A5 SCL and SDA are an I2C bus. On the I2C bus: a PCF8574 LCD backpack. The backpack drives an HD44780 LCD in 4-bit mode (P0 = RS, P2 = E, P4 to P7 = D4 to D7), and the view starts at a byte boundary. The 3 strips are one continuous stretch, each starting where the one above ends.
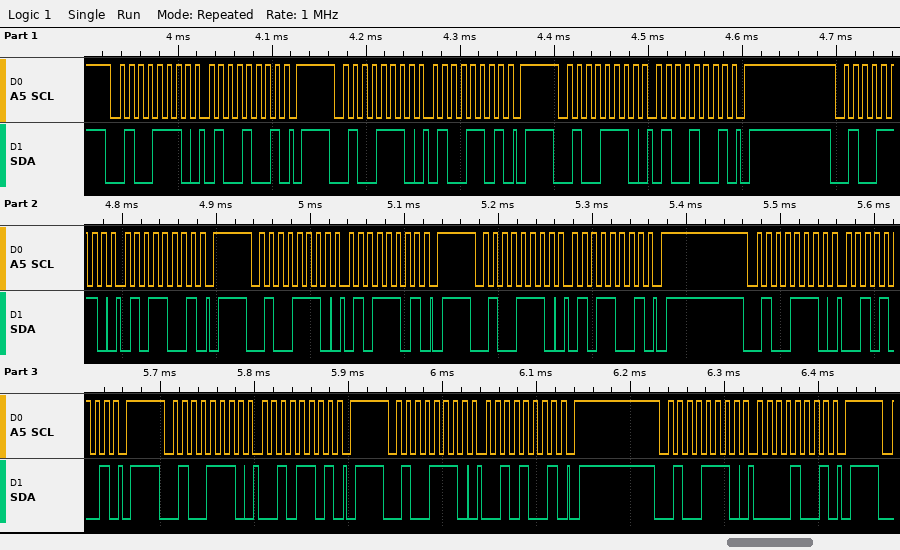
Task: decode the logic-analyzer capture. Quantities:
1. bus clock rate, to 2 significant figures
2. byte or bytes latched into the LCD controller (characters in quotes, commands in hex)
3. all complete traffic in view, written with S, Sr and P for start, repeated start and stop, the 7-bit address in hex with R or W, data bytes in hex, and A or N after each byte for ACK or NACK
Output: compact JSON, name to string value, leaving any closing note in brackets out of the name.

{"bus clock rate, to 2 significant figures": "100 kHz", "byte or bytes latched into the LCD controller": "'E'", "all complete traffic in view, written with S, Sr and P for start, repeated start and stop, the 7-bit address in hex with R or W, data bytes in hex, and A or N after each byte for ACK or NACK": "S 27W A 49 A P S 27W A 4D A P S 27W A 49 A P S 27W A 59 A P S 27W A 5D A P S 27W A 59 A P S 27W A 29 A P S 27W A 2D A P S 27W A 29 A P S 27W A 09 A P"}
